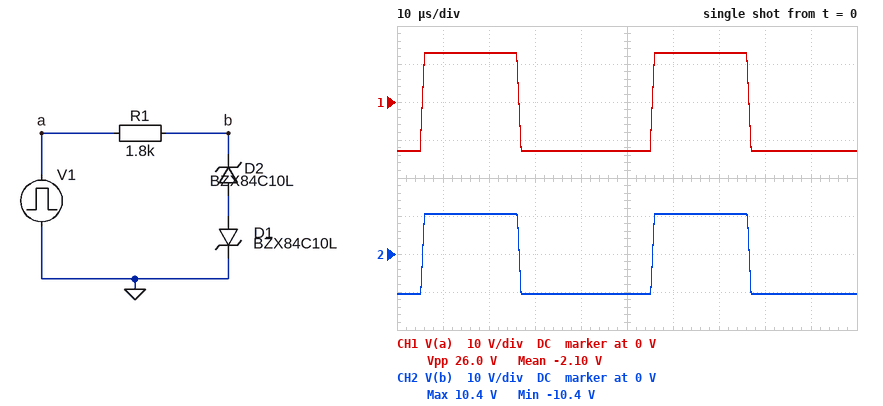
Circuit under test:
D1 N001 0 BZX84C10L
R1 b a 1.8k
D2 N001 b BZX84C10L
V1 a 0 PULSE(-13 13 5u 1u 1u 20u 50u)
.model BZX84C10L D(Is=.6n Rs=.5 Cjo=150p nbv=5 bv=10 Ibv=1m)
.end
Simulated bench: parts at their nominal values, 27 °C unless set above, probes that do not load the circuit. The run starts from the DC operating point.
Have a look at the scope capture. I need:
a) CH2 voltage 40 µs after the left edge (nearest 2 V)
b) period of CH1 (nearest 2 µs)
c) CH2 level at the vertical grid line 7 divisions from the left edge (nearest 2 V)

-10 V
50 µs
10 V
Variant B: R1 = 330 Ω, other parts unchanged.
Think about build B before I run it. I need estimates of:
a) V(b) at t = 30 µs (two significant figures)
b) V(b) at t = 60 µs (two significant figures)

-11 V
11 V
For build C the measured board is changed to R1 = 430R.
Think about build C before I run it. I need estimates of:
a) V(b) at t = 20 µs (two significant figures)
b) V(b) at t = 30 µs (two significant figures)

11 V
-11 V
